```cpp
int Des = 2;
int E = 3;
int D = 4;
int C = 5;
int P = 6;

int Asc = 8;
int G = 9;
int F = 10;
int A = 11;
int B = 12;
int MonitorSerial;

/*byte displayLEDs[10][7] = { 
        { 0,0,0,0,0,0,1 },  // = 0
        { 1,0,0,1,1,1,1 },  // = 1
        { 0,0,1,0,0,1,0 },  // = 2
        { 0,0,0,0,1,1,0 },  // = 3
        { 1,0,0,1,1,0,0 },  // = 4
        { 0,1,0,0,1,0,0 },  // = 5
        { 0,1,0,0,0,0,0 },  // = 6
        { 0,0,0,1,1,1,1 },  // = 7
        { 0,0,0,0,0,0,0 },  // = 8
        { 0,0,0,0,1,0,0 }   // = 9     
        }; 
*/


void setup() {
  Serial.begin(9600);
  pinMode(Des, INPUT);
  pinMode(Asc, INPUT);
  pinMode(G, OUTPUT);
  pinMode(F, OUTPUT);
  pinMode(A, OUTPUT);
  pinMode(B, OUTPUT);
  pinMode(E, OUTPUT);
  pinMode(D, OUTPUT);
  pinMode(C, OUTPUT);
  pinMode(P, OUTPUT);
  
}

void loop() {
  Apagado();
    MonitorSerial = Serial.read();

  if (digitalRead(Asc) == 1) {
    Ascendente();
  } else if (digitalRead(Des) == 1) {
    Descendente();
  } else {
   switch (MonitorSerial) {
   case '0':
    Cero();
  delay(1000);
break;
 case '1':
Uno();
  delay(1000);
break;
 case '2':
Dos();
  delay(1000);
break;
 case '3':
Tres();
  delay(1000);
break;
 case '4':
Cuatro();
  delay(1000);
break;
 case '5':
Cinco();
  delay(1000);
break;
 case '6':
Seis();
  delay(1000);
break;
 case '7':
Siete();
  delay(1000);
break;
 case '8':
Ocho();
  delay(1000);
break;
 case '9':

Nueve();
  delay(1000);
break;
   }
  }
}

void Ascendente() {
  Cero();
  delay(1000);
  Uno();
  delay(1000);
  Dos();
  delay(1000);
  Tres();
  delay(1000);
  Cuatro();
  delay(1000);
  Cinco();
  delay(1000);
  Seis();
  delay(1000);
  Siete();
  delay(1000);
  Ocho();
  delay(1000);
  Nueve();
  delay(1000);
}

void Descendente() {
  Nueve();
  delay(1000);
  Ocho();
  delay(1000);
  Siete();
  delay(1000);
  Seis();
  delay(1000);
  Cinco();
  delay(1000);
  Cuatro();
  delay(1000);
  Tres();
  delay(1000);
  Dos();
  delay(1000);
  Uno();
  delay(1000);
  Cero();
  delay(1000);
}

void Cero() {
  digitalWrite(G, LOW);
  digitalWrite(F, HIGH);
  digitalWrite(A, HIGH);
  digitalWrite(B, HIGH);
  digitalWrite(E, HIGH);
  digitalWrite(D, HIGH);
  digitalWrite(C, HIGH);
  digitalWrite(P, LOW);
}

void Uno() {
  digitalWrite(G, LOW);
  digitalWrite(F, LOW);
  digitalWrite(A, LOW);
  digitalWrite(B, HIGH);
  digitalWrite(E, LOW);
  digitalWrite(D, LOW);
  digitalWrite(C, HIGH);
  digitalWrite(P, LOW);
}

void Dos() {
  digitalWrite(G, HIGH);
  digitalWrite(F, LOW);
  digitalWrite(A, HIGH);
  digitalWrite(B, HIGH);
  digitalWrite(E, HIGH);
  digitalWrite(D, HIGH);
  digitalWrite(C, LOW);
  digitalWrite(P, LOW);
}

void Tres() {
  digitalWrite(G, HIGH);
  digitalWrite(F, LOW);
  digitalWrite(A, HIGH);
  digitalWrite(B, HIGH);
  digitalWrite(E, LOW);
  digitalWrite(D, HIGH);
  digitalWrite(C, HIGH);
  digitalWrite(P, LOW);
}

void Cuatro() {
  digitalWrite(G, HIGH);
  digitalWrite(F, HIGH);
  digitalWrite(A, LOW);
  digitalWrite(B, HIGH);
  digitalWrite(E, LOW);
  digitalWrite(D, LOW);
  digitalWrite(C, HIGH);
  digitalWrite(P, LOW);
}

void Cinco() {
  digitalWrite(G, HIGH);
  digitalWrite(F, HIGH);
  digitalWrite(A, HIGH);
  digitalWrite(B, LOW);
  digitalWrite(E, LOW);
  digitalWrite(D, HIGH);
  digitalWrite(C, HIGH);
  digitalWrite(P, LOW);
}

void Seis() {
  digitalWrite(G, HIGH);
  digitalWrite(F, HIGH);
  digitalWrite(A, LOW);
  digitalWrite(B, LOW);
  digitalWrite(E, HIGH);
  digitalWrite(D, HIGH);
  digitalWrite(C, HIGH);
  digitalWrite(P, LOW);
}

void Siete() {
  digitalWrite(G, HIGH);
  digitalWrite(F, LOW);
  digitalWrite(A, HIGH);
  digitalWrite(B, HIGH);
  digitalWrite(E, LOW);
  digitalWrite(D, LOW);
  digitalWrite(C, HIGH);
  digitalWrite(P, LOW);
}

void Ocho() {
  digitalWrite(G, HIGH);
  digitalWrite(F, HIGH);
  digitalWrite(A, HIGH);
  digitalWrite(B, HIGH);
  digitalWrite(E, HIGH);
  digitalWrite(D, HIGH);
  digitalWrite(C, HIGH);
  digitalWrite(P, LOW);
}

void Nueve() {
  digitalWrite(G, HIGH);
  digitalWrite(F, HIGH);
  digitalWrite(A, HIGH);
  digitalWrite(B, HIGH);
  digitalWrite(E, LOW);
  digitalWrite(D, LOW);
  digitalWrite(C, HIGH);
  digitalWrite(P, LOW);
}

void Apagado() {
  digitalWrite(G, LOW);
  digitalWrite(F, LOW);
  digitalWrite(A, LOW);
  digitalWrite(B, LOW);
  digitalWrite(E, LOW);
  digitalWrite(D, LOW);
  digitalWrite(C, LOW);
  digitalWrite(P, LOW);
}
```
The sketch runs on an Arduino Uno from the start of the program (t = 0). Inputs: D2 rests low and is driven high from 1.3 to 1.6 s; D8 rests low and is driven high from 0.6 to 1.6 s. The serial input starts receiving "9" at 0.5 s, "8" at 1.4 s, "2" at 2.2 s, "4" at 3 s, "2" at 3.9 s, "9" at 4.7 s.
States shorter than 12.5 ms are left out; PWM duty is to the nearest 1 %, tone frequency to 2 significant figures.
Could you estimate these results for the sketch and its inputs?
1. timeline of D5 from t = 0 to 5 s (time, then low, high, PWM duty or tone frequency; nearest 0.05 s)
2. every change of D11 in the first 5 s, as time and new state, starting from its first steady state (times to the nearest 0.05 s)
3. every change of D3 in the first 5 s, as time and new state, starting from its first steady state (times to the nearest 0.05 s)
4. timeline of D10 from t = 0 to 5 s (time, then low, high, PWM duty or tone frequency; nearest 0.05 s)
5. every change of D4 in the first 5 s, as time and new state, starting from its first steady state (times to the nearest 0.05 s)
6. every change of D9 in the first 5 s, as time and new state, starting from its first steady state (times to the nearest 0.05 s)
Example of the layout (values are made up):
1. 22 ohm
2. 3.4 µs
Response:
1. 0 s low; 0.5 s high; 3.5 s low; 4.5 s high
2. 0 s low; 0.5 s high; 2.5 s low; 3.5 s high
3. 0 s low; 1.5 s high; 2.5 s low; 3.5 s high; 4.5 s low
4. 0 s low; 0.5 s high; 2.5 s low
5. 0 s low; 1.5 s high; 2.5 s low; 3.5 s high
6. 0 s low; 0.5 s high; 1.5 s low; 3.5 s high
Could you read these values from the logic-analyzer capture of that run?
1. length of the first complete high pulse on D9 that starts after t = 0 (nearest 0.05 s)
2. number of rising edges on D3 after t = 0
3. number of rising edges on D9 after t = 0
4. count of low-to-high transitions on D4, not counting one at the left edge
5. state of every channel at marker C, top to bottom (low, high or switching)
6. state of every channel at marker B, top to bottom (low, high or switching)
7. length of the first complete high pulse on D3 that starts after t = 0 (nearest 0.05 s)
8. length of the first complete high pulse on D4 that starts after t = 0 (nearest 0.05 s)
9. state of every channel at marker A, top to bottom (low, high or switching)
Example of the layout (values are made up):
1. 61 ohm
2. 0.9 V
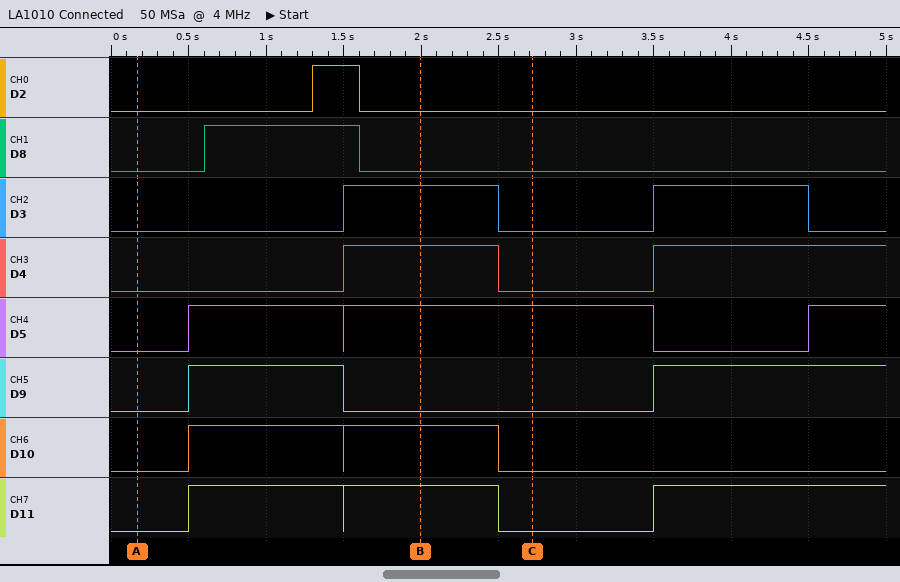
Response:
1. 1.00 s
2. 2
3. 2
4. 2
5. D2 low, D8 low, D3 low, D4 low, D5 high, D9 low, D10 low, D11 low
6. D2 low, D8 low, D3 high, D4 high, D5 high, D9 low, D10 high, D11 high
7. 1.00 s
8. 1.00 s
9. D2 low, D8 low, D3 low, D4 low, D5 low, D9 low, D10 low, D11 low
